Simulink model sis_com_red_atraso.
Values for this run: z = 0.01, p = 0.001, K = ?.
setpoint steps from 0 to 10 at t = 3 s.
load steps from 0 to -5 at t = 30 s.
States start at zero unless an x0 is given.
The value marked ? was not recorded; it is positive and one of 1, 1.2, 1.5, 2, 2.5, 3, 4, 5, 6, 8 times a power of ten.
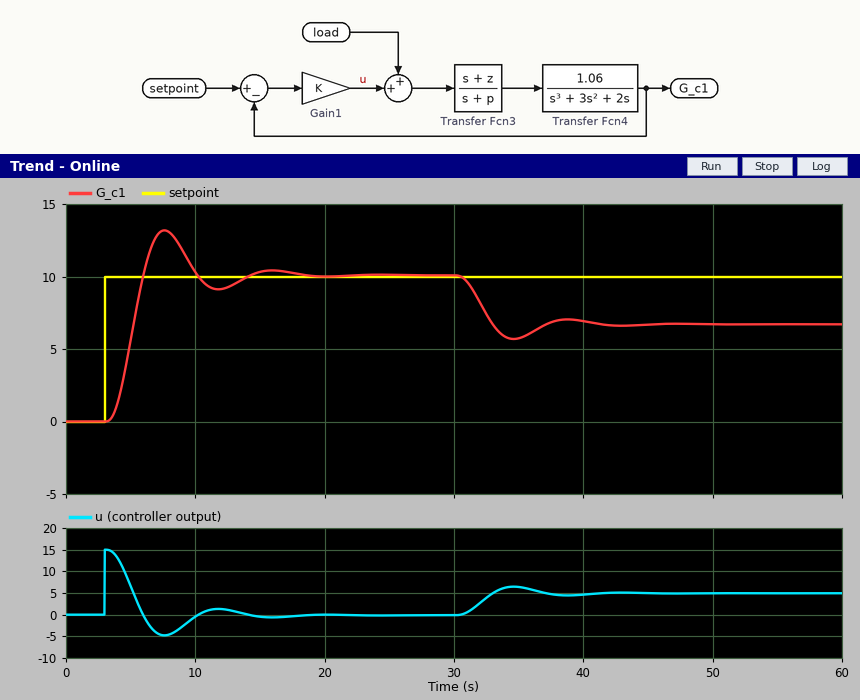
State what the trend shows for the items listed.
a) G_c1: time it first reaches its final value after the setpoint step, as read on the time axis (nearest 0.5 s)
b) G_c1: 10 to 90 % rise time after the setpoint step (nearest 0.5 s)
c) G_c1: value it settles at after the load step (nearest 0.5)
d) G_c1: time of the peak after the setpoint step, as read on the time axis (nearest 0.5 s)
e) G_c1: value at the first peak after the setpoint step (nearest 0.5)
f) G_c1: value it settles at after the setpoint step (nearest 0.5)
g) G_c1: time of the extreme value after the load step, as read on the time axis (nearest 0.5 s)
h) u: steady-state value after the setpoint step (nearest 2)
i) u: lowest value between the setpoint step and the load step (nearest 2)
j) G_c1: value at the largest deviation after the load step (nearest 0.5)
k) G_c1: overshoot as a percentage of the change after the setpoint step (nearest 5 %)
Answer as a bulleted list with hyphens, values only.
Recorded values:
- 6.0 s
- 2.0 s
- 6.5
- 7.5 s
- 13.0
- 10.0
- 34.5 s
- 0
- -4
- 5.5
- 30 %
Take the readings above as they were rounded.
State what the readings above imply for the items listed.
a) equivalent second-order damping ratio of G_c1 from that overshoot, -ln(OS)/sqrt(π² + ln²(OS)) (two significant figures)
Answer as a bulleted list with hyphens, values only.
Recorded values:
- 0.36
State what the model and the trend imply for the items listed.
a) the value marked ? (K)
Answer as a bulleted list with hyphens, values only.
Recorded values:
- 1.5
